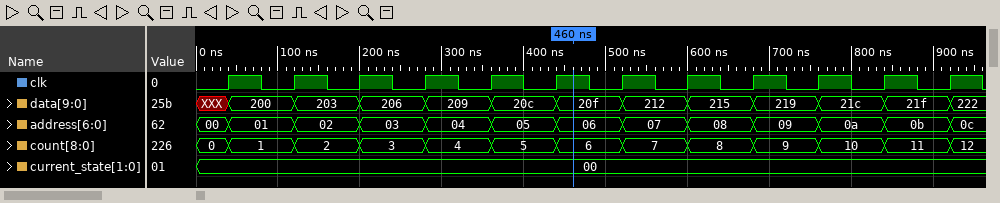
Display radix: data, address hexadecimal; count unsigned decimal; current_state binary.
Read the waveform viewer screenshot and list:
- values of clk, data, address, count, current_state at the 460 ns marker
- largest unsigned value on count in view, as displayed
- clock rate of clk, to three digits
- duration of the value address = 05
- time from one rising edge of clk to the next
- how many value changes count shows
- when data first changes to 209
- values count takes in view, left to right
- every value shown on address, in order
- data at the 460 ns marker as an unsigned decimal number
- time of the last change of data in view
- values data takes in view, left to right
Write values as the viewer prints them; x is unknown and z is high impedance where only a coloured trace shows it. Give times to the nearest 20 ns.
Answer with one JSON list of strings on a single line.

["clk=1, data=20f, address=06, count=6, current_state=00", "12", "12.5 MHz", "80 ns", "80 ns", "12", "280 ns", "0, 1, 2, 3, 4, 5, 6, 7, 8, 9, 10, 11, 12", "00, 01, 02, 03, 04, 05, 06, 07, 08, 09, 0a, 0b, 0c", "527", "920 ns", "XXX, 200, 203, 206, 209, 20c, 20f, 212, 215, 219, 21c, 21f, 222"]
